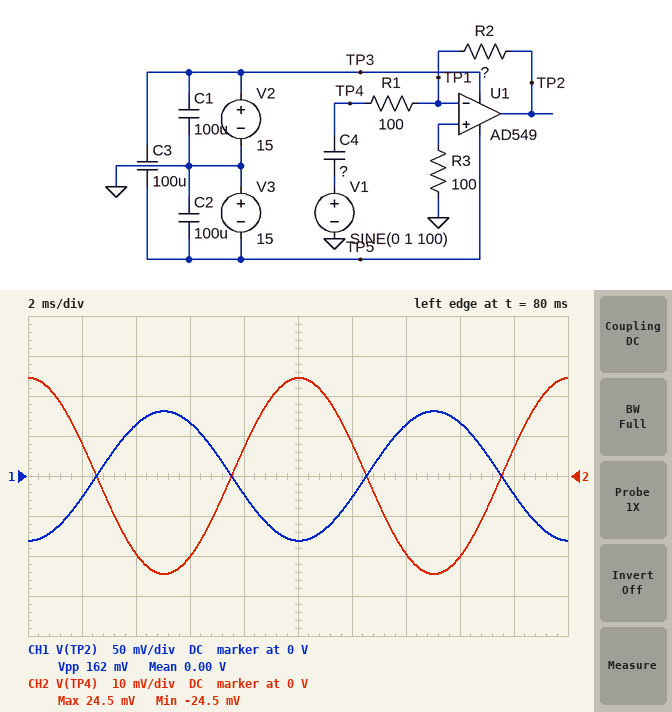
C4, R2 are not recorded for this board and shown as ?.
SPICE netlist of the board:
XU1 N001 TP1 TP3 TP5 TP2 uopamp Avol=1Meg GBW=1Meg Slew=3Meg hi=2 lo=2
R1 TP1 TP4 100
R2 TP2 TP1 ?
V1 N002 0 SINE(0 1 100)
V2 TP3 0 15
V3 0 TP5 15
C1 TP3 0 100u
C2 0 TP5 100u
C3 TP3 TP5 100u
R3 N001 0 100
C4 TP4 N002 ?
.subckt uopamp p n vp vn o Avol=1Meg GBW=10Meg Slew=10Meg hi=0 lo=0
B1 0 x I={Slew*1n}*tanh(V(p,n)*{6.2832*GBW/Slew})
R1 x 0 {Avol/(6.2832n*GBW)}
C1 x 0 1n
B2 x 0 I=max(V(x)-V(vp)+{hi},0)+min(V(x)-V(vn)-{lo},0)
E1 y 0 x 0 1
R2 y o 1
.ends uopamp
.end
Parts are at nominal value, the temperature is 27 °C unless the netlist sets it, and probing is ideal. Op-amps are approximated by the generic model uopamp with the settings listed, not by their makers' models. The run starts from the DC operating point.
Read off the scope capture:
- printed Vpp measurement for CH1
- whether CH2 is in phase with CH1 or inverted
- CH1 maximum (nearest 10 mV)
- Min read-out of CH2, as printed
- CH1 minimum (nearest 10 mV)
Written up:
162 mV
inverted
80 mV
-24.5 mV
-80 mV
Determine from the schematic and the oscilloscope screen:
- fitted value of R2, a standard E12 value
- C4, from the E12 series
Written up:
330 Ω
390 nF
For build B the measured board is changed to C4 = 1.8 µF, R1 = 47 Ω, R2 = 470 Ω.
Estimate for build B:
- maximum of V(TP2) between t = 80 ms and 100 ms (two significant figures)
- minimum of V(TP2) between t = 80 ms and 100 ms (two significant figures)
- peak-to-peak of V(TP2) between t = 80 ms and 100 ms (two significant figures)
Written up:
530 mV
-530 mV
1.1 V
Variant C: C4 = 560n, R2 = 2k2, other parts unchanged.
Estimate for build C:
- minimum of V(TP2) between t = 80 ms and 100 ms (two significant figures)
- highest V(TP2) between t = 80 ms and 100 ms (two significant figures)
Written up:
-770 mV
770 mV
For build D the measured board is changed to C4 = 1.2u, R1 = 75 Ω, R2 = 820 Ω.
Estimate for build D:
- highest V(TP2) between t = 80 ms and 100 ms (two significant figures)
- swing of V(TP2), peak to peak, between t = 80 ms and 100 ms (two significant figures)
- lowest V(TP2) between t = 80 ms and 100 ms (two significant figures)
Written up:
620 mV
1.2 V
-620 mV
